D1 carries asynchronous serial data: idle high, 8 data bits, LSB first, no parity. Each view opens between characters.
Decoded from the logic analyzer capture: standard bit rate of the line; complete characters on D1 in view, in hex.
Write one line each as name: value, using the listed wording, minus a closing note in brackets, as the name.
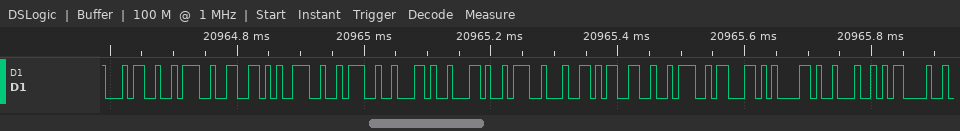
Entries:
standard bit rate of the line: 115200 baud
complete characters on D1 in view, in hex: 34, 3A, 66, 39, 3A, 62, 62, 3A, 64, 33, 3A, 63, 61, 22, 0D
